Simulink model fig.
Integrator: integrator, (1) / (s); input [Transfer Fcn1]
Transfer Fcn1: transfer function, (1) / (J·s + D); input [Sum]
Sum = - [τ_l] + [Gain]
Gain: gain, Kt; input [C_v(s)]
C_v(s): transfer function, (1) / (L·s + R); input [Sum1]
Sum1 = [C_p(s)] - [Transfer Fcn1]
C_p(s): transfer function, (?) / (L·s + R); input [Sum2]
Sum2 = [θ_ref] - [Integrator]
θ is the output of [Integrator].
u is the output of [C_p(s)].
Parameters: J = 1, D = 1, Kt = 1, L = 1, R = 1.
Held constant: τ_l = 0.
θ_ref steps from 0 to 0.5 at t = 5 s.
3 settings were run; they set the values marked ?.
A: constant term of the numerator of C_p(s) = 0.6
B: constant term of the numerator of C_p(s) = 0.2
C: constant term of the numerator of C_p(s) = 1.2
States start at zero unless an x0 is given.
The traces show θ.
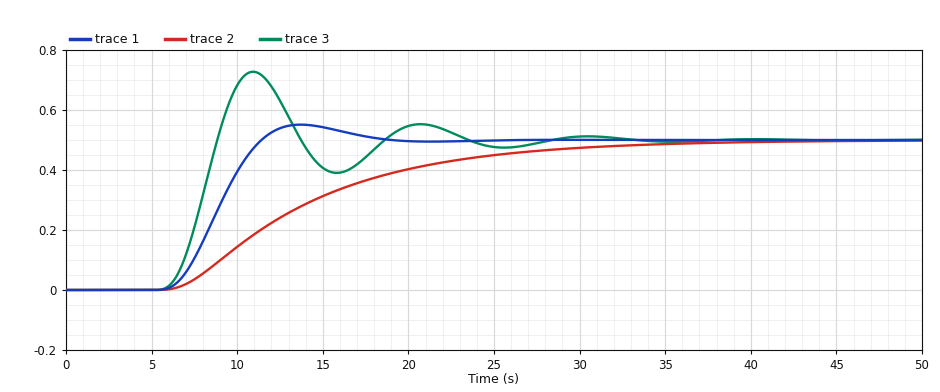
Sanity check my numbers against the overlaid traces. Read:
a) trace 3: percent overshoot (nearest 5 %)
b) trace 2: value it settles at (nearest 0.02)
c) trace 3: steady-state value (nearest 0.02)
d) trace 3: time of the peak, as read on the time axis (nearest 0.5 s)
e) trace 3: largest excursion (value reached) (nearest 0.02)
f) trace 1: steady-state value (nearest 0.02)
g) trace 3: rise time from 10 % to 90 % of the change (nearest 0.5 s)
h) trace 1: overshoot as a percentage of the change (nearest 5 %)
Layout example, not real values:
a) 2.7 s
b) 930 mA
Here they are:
a) 45 %
b) 0.50
c) 0.50
d) 11.0 s
e) 0.72
f) 0.50
g) 2.0 s
h) 10 %
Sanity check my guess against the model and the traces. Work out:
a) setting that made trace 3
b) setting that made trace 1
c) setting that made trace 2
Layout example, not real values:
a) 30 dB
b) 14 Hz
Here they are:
a) C
b) A
c) B
